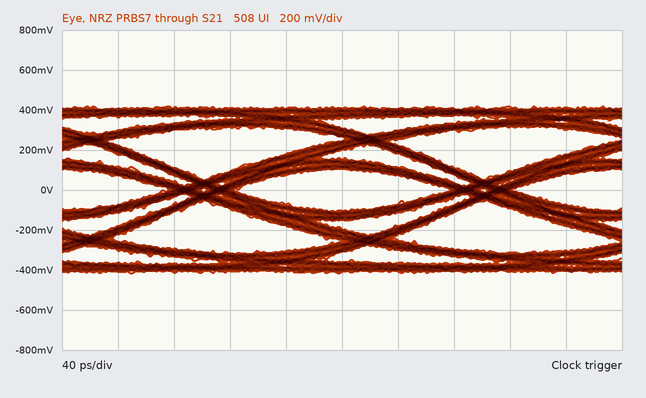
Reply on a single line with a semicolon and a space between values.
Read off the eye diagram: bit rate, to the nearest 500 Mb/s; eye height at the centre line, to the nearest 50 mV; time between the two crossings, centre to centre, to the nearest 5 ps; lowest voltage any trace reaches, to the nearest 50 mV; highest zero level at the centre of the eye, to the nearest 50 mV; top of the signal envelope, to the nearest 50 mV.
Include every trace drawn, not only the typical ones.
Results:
5.0 Gb/s; 200 mV; 200 ps; -400 mV; -100 mV; 400 mV
